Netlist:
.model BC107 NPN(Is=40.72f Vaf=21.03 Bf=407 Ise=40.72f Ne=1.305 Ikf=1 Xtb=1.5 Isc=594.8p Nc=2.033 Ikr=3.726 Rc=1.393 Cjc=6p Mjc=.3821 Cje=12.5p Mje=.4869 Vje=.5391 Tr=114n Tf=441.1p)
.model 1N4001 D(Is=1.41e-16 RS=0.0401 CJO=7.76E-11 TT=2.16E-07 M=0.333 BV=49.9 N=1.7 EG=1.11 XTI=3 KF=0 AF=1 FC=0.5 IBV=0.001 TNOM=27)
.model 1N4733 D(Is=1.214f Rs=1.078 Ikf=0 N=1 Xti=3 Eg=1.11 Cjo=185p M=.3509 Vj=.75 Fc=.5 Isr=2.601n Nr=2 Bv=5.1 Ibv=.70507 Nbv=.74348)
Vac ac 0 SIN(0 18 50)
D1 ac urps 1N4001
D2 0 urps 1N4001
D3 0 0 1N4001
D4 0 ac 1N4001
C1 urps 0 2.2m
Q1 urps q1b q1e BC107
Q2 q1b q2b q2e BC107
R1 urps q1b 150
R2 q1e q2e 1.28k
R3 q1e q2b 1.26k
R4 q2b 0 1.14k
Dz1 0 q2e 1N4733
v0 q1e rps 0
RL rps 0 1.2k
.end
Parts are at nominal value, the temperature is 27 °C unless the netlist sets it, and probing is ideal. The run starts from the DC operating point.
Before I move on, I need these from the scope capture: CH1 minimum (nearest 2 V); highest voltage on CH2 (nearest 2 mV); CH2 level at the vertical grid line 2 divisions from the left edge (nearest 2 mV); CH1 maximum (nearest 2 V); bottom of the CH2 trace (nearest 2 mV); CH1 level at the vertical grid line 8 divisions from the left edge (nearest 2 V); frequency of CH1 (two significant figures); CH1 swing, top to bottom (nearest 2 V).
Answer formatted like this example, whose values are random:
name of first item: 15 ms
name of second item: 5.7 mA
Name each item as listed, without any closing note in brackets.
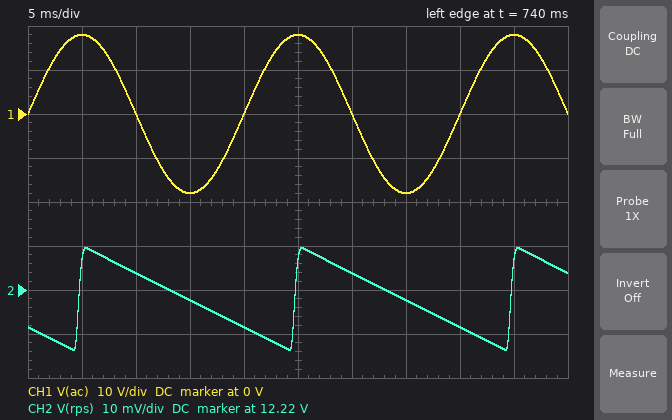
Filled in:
CH1 minimum: -18 V
highest voltage on CH2: 12.230 V
CH2 level at the vertical grid line 2 divisions from the left edge: 12.224 V
CH1 maximum: 18 V
bottom of the CH2 trace: 12.206 V
CH1 level at the vertical grid line 8 divisions from the left edge: 0 V
frequency of CH1: 50 Hz
CH1 swing, top to bottom: 36 V
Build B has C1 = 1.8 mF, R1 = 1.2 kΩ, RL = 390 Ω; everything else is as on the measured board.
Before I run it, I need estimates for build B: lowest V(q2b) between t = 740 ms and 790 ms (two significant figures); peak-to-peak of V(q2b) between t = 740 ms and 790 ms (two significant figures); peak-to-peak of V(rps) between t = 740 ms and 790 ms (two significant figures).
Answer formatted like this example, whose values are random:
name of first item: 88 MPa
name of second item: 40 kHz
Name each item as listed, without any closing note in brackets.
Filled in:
lowest V(q2b) between t = 740 ms and 790 ms: 5.7 V
peak-to-peak of V(q2b) between t = 740 ms and 790 ms: 4.7 mV
peak-to-peak of V(rps) between t = 740 ms and 790 ms: 12 mV
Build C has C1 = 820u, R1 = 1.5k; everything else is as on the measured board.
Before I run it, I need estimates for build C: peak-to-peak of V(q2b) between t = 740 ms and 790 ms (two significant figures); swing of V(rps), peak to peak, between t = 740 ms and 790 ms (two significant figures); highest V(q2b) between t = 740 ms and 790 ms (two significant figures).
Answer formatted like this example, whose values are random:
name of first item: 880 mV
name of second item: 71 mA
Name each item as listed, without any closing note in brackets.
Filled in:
peak-to-peak of V(q2b) between t = 740 ms and 790 ms: 5.0 mV
swing of V(rps), peak to peak, between t = 740 ms and 790 ms: 12 mV
highest V(q2b) between t = 740 ms and 790 ms: 5.7 V
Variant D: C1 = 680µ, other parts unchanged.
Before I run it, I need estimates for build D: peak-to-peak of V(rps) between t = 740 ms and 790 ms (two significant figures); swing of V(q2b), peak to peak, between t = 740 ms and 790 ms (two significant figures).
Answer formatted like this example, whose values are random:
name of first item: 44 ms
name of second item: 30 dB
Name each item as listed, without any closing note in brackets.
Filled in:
peak-to-peak of V(rps) between t = 740 ms and 790 ms: 73 mV
swing of V(q2b), peak to peak, between t = 740 ms and 790 ms: 22 mV
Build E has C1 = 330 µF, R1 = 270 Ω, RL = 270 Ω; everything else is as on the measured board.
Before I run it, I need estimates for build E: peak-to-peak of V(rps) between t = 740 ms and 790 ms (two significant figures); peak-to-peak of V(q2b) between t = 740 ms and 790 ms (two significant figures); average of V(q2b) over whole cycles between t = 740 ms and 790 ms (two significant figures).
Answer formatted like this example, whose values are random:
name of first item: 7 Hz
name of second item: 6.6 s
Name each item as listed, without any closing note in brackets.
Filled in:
peak-to-peak of V(rps) between t = 740 ms and 790 ms: 230 mV
peak-to-peak of V(q2b) between t = 740 ms and 790 ms: 84 mV
average of V(q2b) over whole cycles between t = 740 ms and 790 ms: 5.7 V
